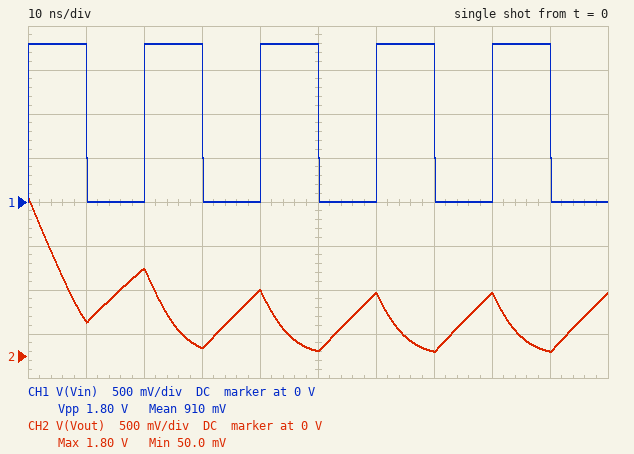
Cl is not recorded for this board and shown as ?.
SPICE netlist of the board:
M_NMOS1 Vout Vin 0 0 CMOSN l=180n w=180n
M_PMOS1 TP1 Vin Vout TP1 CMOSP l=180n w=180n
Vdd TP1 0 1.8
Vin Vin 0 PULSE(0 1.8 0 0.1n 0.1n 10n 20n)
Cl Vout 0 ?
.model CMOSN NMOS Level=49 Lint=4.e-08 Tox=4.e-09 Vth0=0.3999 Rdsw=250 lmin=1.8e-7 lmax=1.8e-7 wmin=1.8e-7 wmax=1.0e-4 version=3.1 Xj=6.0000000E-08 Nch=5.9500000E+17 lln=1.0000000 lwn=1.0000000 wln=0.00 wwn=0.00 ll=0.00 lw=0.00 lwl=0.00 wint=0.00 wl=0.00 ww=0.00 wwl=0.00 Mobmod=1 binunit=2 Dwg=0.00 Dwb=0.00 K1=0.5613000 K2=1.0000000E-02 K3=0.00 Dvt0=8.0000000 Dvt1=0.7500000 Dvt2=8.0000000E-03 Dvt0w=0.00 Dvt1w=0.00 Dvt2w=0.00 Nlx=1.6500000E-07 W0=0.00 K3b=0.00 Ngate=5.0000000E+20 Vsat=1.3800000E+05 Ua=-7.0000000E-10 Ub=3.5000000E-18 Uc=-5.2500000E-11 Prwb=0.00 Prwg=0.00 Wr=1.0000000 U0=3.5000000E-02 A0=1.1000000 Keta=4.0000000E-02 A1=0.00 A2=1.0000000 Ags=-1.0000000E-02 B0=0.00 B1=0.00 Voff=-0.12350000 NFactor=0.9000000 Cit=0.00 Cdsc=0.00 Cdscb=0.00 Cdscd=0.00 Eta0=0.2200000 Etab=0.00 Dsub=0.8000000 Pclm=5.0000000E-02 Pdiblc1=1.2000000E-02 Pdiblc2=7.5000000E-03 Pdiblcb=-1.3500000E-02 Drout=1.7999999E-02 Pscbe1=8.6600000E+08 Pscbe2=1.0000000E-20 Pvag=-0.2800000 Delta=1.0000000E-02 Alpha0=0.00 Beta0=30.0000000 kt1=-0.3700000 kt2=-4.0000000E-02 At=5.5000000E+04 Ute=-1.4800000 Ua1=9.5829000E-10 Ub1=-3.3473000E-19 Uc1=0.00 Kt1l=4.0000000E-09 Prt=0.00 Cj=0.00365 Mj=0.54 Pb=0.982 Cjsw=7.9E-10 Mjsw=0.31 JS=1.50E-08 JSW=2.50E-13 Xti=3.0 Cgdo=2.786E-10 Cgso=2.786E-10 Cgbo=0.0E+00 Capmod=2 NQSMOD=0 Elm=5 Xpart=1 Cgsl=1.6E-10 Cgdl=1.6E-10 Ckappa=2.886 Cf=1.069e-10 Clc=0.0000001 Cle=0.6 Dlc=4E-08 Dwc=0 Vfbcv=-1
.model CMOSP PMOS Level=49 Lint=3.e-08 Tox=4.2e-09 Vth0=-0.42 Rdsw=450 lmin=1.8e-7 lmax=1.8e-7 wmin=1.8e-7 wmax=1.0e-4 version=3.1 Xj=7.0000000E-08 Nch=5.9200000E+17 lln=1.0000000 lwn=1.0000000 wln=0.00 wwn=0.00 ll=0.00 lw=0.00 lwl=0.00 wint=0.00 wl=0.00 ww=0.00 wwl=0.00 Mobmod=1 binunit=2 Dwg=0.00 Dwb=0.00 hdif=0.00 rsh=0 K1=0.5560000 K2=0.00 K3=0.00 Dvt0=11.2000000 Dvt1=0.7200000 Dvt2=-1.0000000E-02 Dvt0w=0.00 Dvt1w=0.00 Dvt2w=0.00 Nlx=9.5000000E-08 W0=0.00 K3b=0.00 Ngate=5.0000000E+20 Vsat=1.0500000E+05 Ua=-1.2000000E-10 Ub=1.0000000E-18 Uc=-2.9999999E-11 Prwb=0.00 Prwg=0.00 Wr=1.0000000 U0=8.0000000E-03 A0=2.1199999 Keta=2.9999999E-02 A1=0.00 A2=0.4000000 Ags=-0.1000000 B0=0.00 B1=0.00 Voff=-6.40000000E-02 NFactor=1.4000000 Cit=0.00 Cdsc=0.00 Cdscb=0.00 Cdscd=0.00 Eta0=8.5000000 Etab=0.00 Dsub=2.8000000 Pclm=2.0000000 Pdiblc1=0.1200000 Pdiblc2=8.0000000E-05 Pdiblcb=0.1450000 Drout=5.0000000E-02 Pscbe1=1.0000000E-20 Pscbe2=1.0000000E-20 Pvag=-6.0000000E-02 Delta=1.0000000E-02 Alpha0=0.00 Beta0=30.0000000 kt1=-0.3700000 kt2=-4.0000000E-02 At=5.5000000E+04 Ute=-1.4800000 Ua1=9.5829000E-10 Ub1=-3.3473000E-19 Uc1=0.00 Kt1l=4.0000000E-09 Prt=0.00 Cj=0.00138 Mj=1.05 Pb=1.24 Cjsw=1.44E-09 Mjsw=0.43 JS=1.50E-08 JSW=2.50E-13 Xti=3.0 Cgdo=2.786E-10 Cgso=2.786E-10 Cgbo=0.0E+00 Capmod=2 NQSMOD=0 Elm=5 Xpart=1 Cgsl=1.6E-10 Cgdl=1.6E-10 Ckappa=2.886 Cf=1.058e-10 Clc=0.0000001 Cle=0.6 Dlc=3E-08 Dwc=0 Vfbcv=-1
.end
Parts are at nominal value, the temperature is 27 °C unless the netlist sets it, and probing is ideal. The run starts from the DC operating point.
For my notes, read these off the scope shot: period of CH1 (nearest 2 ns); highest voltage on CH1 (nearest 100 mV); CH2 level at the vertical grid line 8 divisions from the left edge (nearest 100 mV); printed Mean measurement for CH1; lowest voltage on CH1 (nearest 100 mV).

20 ns
1.8 V
700 mV
910 mV
0 V
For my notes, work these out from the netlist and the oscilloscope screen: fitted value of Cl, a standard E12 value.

820 fF
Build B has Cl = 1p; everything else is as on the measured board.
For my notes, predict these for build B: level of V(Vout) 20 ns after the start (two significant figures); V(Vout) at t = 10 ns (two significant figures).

1.1 V
590 mV
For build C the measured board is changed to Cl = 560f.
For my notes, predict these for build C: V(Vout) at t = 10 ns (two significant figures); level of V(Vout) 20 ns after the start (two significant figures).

110 mV
1.0 V
